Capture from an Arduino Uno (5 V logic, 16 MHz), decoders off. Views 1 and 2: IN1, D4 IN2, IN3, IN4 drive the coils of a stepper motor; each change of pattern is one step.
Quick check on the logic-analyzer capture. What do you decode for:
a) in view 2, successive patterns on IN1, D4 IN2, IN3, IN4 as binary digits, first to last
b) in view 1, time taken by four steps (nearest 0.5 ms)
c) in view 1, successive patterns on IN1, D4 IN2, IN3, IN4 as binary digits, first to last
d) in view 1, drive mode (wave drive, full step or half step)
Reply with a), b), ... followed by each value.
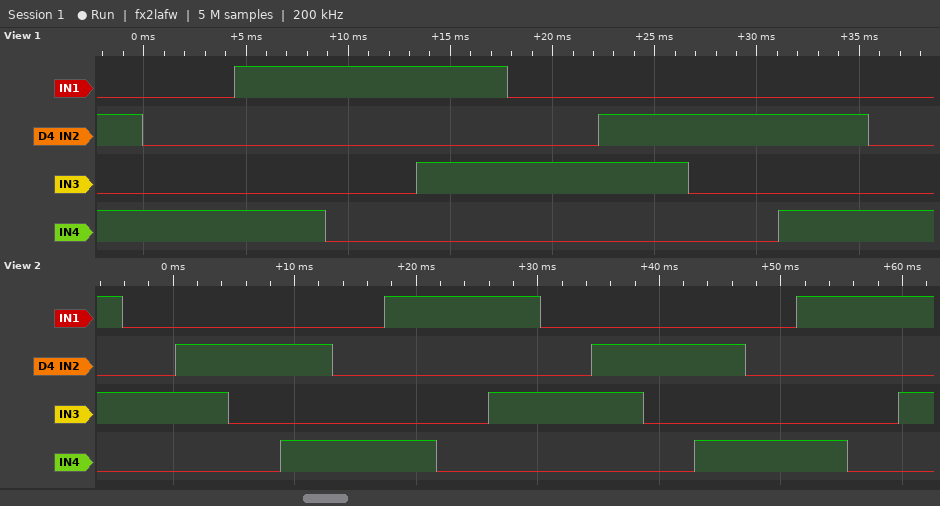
a) 1010 0010 0110 0100 0101 0001 1001 1000 1010 0010 0110 0100 0101 0001 1001 1000 1010
b) 18.0 ms
c) 0101 0001 1001 1000 1010 0010 0110 0100 0101 0001
d) half step
